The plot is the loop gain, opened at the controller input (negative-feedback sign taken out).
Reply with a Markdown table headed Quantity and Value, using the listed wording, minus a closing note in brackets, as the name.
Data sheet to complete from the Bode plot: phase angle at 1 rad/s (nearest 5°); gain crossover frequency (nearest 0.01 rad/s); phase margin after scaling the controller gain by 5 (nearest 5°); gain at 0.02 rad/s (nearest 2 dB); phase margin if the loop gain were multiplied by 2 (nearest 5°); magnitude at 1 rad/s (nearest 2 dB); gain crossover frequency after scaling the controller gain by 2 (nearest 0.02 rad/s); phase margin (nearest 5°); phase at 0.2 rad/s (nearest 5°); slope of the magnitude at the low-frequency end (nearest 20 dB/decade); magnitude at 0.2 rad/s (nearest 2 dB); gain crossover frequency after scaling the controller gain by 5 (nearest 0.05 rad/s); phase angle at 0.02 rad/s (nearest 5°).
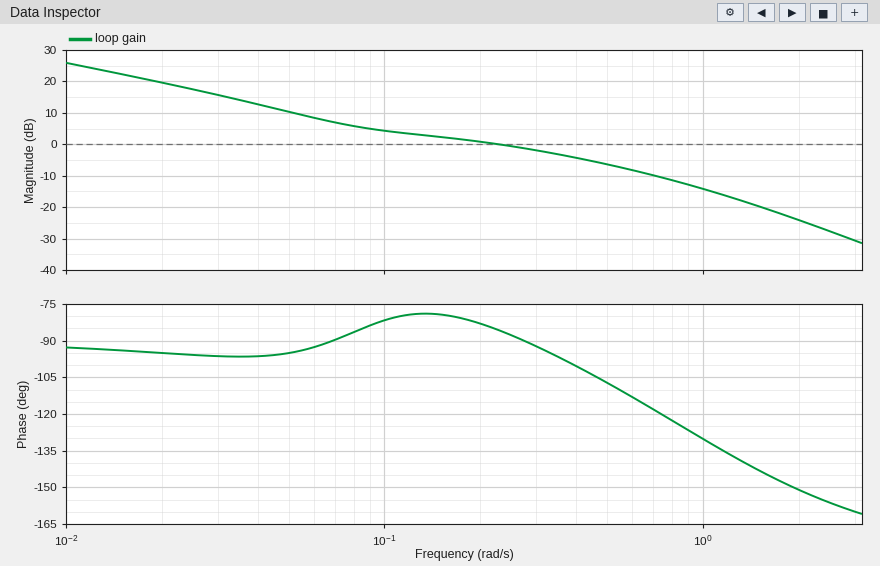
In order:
| Quantity | Value |
|---|---|
| phase angle at 1 rad/s | -130° |
| gain crossover frequency | 0.23 rad/s |
| phase margin after scaling the controller gain by 5 | 50° |
| gain at 0.02 rad/s | 20 dB |
| phase margin if the loop gain were multiplied by 2 | 75° |
| magnitude at 1 rad/s | -14 dB |
| gain crossover frequency after scaling the controller gain by 2 | 0.48 rad/s |
| phase margin | 95° |
| phase at 0.2 rad/s | -85° |
| slope of the magnitude at the low-frequency end | -20 dB/decade |
| magnitude at 0.2 rad/s | 0 dB |
| gain crossover frequency after scaling the controller gain by 5 | 1.00 rad/s |
| phase angle at 0.02 rad/s | -95° |
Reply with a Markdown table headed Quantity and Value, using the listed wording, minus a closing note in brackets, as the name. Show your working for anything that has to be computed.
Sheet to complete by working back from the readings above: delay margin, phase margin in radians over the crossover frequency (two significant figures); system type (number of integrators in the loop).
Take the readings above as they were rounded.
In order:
| Quantity | Value |
|---|---|
| delay margin, phase margin in radians over the crossover frequency | 95 × π / 180 / 0.23 = 7.2 s |
| system type | 1 |
